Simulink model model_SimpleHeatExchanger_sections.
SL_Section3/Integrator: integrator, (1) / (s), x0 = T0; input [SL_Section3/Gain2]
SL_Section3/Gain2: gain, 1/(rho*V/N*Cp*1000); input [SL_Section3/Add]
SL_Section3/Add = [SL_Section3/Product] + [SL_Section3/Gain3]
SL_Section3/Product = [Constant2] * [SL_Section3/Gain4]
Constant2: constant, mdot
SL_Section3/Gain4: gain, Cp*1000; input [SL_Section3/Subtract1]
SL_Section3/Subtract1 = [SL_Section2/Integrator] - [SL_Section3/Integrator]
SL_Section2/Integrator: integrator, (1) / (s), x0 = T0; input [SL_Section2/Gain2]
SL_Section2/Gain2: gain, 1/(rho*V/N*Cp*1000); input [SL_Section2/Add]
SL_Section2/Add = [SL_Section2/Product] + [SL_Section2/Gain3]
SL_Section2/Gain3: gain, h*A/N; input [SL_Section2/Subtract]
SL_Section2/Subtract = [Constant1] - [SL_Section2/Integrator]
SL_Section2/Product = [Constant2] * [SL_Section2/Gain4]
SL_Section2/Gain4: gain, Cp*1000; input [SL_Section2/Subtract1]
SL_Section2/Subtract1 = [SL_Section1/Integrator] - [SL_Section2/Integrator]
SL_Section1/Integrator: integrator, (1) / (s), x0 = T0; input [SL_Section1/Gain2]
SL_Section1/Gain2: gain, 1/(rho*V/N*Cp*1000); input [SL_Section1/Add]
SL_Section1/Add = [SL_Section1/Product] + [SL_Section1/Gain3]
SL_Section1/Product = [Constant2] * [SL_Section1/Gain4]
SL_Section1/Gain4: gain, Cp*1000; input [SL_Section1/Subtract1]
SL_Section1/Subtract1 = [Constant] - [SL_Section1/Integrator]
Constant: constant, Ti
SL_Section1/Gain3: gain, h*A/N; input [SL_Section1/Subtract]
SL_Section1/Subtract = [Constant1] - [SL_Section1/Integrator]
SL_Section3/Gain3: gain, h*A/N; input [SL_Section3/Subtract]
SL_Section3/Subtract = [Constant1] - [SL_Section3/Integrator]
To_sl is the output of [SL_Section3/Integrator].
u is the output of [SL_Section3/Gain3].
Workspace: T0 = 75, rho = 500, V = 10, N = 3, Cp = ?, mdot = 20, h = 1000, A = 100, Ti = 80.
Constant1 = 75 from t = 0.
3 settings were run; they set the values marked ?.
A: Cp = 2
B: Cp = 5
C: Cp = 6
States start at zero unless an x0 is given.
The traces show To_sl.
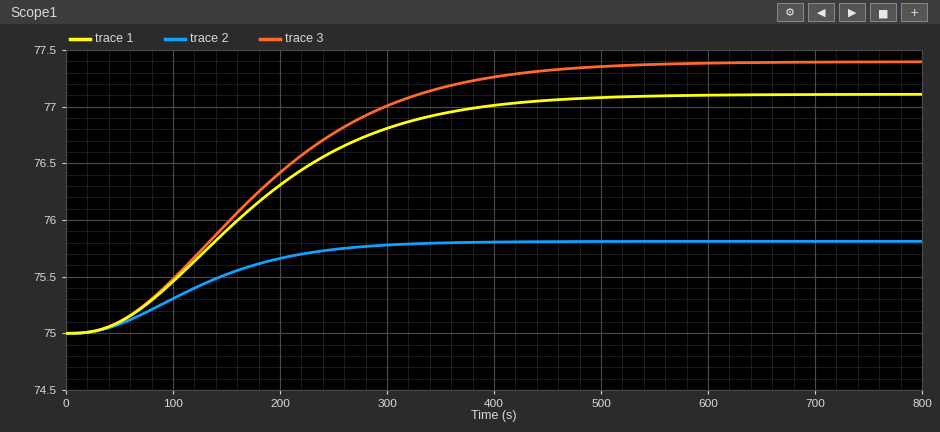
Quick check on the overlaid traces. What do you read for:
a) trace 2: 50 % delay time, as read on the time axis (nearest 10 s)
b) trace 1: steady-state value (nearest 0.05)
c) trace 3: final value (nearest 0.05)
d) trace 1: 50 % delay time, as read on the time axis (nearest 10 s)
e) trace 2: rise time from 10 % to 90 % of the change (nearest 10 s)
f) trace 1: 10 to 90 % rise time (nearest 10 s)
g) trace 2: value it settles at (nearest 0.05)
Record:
120 s
77.10
77.40
170 s
190 s
260 s
75.80
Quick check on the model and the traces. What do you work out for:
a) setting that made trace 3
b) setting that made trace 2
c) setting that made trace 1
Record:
C
A
B
